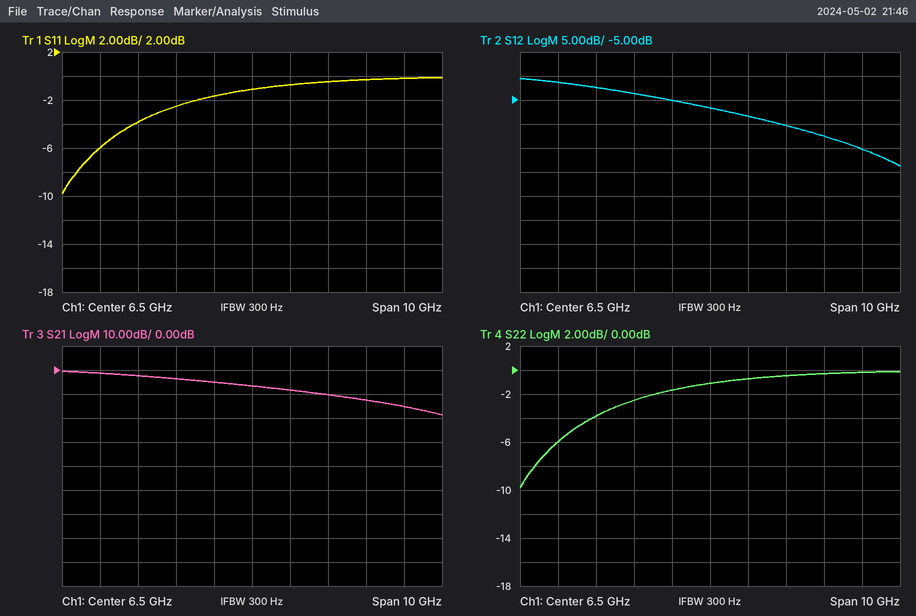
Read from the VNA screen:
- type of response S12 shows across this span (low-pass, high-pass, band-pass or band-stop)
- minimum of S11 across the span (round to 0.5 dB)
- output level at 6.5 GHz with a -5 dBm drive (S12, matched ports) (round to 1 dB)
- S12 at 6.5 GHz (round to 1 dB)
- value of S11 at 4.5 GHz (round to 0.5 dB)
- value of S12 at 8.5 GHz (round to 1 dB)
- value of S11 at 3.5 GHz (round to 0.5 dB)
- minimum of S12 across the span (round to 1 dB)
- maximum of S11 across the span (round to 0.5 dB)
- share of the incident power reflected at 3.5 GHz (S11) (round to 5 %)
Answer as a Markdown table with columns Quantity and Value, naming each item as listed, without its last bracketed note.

| Quantity | Value |
|---|---|
| type of response S12 shows across this span | low-pass |
| minimum of S11 across the span | -10.0 dB |
| output level at 6.5 GHz with a -5 dBm drive (S12, matched ports) | -12 dBm |
| S12 at 6.5 GHz | -7 dB |
| value of S11 at 4.5 GHz | -2.5 dB |
| value of S12 at 8.5 GHz | -10 dB |
| value of S11 at 3.5 GHz | -4.0 dB |
| minimum of S12 across the span | -19 dB |
| maximum of S11 across the span | 0.0 dB |
| share of the incident power reflected at 3.5 GHz (S11) | 40 % |
